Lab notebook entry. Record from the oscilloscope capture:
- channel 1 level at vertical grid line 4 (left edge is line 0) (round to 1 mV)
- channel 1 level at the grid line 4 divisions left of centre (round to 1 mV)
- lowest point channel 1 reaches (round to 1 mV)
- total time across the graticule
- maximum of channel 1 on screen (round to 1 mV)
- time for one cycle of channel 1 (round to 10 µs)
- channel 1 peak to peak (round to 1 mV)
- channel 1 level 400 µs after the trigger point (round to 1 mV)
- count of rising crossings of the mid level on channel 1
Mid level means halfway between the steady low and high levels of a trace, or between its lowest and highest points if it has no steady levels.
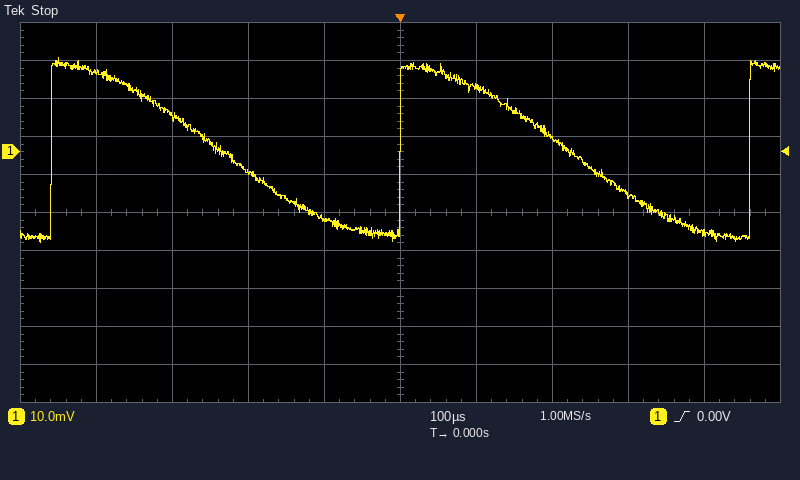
-17 mV
21 mV
-24 mV
1 ms
25 mV
460 µs
49 mV
-21 mV
3
